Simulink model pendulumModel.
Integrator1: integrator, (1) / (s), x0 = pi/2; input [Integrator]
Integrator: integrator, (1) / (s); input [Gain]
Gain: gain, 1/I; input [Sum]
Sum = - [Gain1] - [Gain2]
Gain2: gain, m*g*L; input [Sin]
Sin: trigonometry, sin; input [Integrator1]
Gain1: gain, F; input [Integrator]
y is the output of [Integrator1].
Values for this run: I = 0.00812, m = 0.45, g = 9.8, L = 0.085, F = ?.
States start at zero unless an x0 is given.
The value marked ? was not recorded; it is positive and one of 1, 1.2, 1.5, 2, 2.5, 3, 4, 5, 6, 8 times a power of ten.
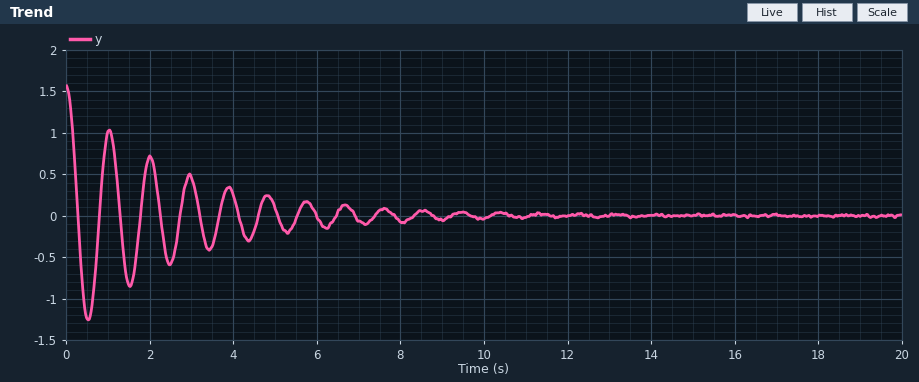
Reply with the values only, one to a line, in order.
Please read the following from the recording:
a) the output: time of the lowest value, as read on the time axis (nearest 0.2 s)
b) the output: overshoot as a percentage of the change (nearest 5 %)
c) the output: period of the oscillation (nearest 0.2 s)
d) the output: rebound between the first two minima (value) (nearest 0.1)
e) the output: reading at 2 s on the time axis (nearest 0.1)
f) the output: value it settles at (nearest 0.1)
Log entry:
0.6 s
80 %
1.0 s
1.0
0.7
0.0
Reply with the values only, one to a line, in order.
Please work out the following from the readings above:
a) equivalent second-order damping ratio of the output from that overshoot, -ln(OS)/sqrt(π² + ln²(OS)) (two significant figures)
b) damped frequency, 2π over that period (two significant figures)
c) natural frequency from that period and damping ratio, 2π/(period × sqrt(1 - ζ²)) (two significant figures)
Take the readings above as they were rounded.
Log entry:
0.071
6.3 rad/s
6.3 rad/s
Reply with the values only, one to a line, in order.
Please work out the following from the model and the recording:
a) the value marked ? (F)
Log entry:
0.006
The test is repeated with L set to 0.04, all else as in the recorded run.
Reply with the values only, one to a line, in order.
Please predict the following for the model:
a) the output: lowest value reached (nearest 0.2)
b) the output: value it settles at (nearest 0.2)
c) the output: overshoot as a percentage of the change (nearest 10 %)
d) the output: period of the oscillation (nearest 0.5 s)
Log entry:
-1.2
0.0
70 %
1.5 s
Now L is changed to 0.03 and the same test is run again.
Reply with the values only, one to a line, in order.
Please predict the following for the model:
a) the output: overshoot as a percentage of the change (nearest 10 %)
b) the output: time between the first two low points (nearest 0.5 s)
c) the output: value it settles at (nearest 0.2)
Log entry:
70 %
1.5 s
0.0
